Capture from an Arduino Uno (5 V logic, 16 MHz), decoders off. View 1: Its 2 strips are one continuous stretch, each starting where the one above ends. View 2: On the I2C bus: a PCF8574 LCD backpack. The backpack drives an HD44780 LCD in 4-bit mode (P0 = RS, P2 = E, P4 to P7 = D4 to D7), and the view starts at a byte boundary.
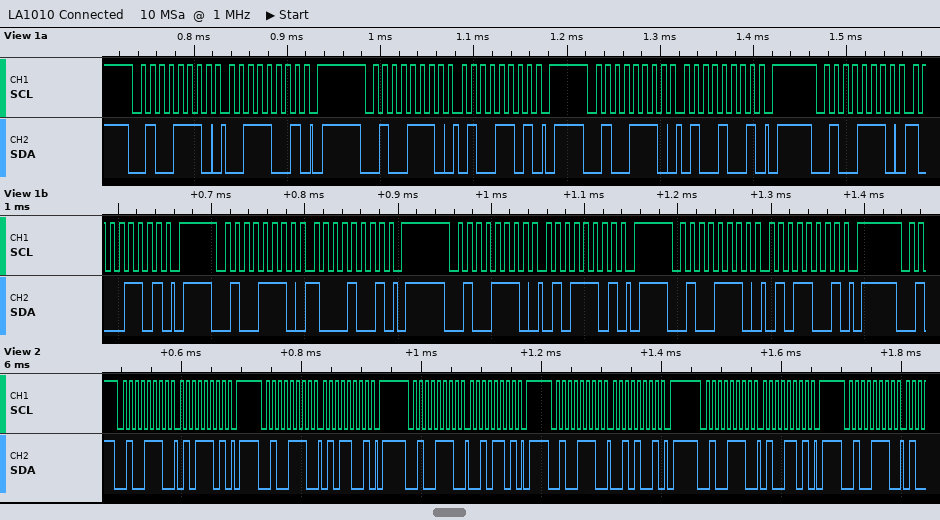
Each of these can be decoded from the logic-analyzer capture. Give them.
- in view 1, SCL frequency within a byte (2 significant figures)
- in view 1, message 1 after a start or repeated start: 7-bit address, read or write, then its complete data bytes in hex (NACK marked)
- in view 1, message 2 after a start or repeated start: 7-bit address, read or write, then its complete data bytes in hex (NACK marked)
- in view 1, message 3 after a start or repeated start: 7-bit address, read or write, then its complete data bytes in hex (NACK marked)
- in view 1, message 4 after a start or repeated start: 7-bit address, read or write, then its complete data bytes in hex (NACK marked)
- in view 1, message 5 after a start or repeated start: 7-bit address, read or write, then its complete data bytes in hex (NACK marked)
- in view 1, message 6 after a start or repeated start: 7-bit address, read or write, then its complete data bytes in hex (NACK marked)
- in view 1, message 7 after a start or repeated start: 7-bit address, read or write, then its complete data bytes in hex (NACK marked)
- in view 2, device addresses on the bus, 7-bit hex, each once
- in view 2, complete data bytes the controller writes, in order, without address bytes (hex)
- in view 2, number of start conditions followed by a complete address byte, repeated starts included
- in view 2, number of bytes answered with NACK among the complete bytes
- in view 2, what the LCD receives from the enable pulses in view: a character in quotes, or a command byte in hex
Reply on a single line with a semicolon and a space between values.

100 kHz; 0x27 write: 39; 0x27 write: 4D; 0x27 write: 49; 0x27 write: 8D; 0x27 write: 89; 0x27 write: 5D; 0x27 write: 59; 0x27; 5D 59 2D 29 4D; 6; 0; 'R'
